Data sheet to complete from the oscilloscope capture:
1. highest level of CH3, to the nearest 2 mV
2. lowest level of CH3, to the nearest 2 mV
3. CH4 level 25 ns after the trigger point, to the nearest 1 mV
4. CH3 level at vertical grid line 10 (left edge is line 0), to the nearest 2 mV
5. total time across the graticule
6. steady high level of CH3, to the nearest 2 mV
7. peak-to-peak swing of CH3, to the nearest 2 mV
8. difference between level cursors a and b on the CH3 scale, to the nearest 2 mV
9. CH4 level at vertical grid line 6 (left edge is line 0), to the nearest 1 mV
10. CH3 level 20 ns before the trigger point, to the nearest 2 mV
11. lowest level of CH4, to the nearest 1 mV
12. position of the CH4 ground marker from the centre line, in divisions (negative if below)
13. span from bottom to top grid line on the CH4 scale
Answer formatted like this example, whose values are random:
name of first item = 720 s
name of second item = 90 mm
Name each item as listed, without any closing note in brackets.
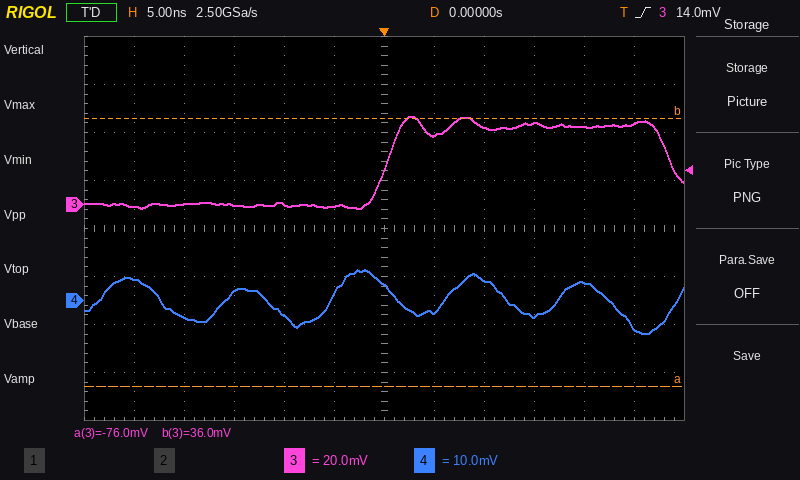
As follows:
highest level of CH3, to the nearest 2 mV = 36 mV
lowest level of CH3, to the nearest 2 mV = -2 mV
CH4 level 25 ns after the trigger point, to the nearest 1 mV = -6 mV
CH3 level at vertical grid line 10 (left edge is line 0), to the nearest 2 mV = 32 mV
total time across the graticule = 60 ns
steady high level of CH3, to the nearest 2 mV = 32 mV
peak-to-peak swing of CH3, to the nearest 2 mV = 38 mV
difference between level cursors a and b on the CH3 scale, to the nearest 2 mV = 112 mV
CH4 level at vertical grid line 6 (left edge is line 0), to the nearest 1 mV = 3 mV
CH3 level 20 ns before the trigger point, to the nearest 2 mV = 0 mV
lowest level of CH4, to the nearest 1 mV = -7 mV
position of the CH4 ground marker from the centre line, in divisions = -1.5 div
span from bottom to top grid line on the CH4 scale = 80 mV
